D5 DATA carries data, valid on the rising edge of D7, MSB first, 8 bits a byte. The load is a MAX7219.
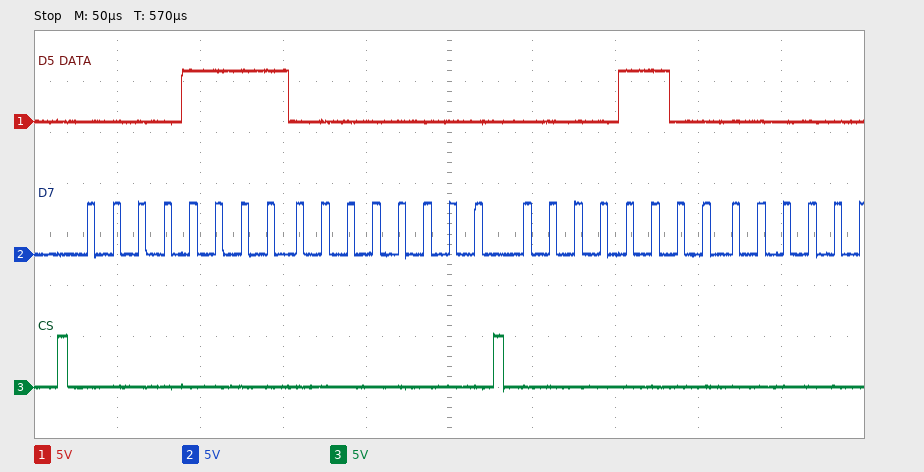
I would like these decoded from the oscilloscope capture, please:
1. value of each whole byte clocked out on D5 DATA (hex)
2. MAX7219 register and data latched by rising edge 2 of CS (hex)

0F 00 0C
register 0xF, data 0x00
